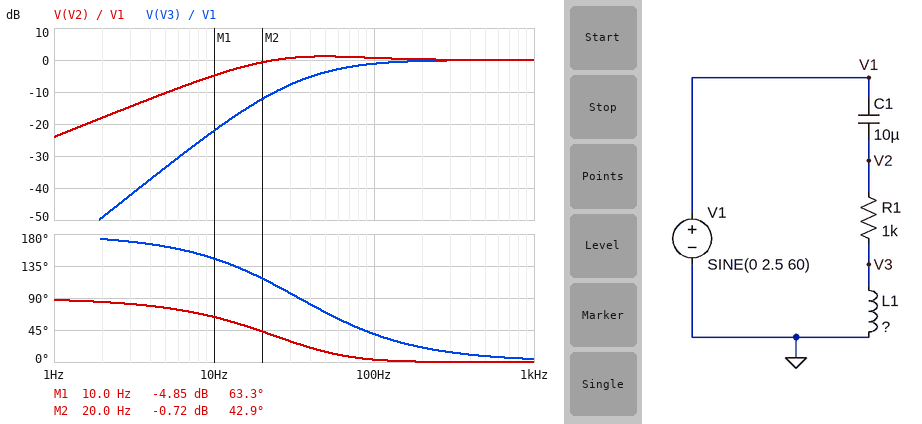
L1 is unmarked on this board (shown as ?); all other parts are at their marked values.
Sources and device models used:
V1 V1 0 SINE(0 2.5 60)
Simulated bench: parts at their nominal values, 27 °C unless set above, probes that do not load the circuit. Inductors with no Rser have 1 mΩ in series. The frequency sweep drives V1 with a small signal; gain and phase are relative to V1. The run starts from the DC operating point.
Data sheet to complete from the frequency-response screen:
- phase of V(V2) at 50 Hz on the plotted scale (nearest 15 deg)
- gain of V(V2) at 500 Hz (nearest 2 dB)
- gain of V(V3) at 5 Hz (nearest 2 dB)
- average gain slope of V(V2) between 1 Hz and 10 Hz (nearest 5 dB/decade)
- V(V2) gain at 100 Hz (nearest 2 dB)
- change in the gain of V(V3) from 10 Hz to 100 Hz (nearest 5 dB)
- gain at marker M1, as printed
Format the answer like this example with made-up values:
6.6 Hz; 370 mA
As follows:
15 deg; 0 dB; -34 dB; 20 dB/decade; 0 dB; 20 dB; -4.85 dB
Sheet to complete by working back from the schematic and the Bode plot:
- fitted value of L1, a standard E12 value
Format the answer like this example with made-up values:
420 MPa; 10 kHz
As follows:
2.2 H
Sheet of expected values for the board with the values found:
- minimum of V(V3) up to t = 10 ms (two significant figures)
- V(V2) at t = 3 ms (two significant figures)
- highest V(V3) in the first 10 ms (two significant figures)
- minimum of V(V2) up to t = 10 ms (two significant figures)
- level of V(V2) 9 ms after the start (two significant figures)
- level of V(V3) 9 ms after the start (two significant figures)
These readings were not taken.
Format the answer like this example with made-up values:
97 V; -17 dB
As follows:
-1.7 V; 2.1 V; 1.1 V; -2.4 V; -1.5 V; -1.7 V
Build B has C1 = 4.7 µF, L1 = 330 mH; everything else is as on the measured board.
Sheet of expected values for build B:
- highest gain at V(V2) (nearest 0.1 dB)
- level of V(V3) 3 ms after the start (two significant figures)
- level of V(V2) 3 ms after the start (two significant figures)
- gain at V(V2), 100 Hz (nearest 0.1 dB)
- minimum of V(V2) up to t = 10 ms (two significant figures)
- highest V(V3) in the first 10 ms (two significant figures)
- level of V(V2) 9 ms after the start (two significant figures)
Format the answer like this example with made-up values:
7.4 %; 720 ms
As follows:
0.4 dB; 57 mV; 1.7 V; 0.1 dB; -2.2 V; 260 mV; -1.8 V
